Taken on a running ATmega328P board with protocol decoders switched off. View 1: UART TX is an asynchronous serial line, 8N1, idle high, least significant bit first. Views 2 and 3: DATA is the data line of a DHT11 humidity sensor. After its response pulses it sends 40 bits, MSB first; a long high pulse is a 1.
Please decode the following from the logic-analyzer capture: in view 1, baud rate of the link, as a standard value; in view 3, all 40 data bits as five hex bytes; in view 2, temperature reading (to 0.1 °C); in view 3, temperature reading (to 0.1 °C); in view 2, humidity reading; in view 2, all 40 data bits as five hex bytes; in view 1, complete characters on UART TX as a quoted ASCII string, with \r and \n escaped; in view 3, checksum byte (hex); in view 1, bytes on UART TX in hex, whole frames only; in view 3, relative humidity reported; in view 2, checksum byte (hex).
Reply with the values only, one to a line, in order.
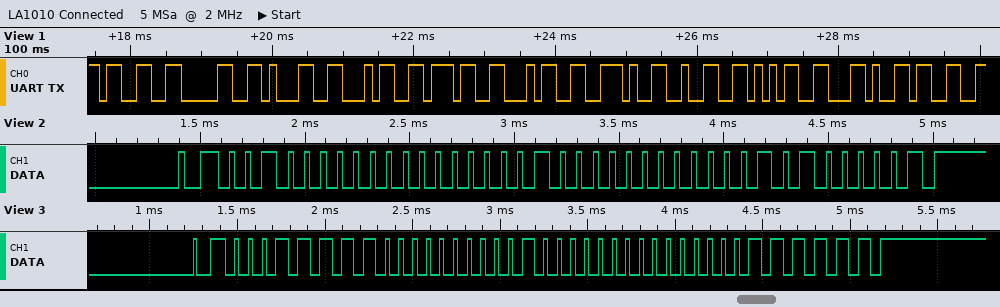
9600 baud
1F 00 20 00 3F
32.1 °C
32.0 °C
32 %
20 00 20 01 41
"301474.25,3"
0x3F
33 30 31 34 37 34 2E 32 35 2C 33
31 %
0x41
